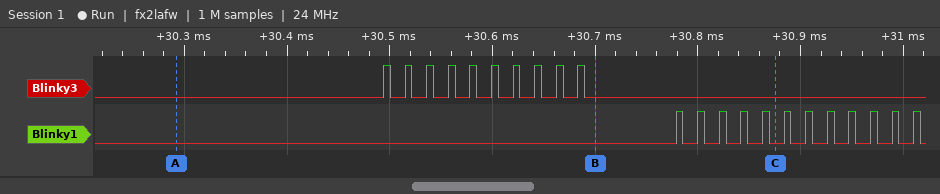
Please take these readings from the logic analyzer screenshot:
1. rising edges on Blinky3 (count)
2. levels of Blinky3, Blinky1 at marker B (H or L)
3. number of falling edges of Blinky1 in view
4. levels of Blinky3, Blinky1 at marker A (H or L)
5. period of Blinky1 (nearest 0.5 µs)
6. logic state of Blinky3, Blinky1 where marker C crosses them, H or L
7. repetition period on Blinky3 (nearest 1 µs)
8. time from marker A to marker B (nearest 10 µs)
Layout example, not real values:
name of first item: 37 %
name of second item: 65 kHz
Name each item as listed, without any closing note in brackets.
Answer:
rising edges on Blinky3: 10
levels of Blinky3, Blinky1 at marker B: Blinky3=L, Blinky1=L
number of falling edges of Blinky1 in view: 12
levels of Blinky3, Blinky1 at marker A: Blinky3=L, Blinky1=L
period of Blinky1: 21 µs
logic state of Blinky3, Blinky1 where marker C crosses them, H or L: Blinky3=L, Blinky1=L
repetition period on Blinky3: 21 µs
time from marker A to marker B: 410 µs
